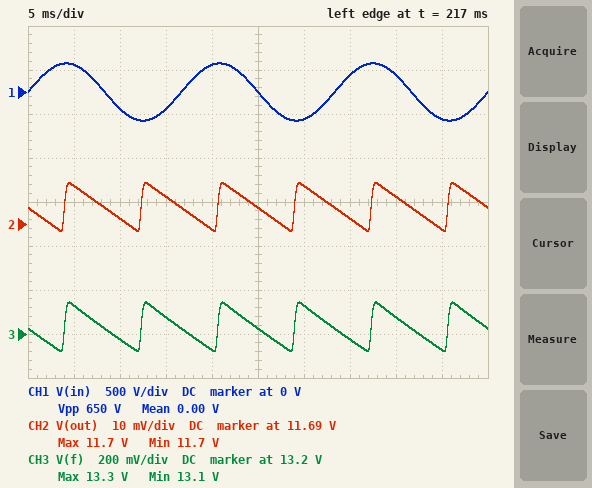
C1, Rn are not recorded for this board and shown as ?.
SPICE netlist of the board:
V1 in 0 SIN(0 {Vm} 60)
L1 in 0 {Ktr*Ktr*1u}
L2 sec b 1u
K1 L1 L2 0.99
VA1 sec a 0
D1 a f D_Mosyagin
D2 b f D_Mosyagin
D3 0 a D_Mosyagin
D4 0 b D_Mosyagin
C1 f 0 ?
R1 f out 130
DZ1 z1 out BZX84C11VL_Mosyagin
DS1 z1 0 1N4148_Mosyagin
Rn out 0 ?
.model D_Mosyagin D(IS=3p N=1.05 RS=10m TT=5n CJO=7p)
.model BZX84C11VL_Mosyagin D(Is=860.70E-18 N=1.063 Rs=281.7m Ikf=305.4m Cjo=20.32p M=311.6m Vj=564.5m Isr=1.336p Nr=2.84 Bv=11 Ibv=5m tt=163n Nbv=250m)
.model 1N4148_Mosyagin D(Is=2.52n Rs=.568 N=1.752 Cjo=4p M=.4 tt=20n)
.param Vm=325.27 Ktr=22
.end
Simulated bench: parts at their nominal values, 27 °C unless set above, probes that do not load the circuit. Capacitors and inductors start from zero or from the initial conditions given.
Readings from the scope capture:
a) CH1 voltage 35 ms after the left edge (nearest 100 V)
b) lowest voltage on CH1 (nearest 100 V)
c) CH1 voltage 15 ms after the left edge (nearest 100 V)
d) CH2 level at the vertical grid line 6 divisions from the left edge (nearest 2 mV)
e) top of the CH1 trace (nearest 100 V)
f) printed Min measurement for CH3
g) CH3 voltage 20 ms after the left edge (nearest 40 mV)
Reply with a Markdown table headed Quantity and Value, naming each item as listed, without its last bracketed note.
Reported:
| Quantity | Value |
|---|---|
| CH1 voltage 35 ms after the left edge | 200 V |
| lowest voltage on CH1 | -300 V |
| CH1 voltage 15 ms after the left edge | -200 V |
| CH2 level at the vertical grid line 6 divisions from the left edge | 11.698 V |
| top of the CH1 trace | 300 V |
| printed Min measurement for CH3 | 13.1 V |
| CH3 voltage 20 ms after the left edge | 13.12 V |
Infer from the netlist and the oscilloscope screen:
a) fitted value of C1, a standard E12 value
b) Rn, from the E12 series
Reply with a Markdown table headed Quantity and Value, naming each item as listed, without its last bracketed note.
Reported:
| Quantity | Value |
|---|---|
| fitted value of C1, a standard E12 value | 390 µF |
| Rn, from the E12 series | 3.9 kΩ |
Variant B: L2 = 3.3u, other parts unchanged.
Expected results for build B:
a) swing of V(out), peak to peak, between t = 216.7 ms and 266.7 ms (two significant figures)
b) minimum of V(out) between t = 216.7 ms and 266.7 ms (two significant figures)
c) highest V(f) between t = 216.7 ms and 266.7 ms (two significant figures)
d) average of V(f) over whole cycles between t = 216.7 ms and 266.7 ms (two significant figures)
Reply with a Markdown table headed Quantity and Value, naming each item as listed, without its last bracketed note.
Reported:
| Quantity | Value |
|---|---|
| swing of V(out), peak to peak, between t = 216.7 ms and 266.7 ms | 19 mV |
| minimum of V(out) between t = 216.7 ms and 266.7 ms | 12 V |
| highest V(f) between t = 216.7 ms and 266.7 ms | 25 V |
| average of V(f) over whole cycles between t = 216.7 ms and 266.7 ms | 24 V |
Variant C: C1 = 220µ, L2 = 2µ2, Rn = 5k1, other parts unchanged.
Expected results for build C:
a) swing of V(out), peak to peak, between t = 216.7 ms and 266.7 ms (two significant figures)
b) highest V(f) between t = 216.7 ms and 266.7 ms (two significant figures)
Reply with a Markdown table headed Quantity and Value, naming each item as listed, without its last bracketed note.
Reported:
| Quantity | Value |
|---|---|
| swing of V(out), peak to peak, between t = 216.7 ms and 266.7 ms | 25 mV |
| highest V(f) between t = 216.7 ms and 266.7 ms | 20 V |
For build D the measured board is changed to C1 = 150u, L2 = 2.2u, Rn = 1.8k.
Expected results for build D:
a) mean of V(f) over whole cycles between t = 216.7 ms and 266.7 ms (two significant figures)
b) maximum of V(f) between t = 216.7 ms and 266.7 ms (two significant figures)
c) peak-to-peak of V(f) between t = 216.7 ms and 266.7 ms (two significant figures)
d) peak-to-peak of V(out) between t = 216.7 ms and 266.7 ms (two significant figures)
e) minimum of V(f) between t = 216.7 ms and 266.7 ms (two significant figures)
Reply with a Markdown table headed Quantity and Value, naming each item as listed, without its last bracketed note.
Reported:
| Quantity | Value |
|---|---|
| mean of V(f) over whole cycles between t = 216.7 ms and 266.7 ms | 19 V |
| maximum of V(f) between t = 216.7 ms and 266.7 ms | 20 V |
| peak-to-peak of V(f) between t = 216.7 ms and 266.7 ms | 2.5 V |
| peak-to-peak of V(out) between t = 216.7 ms and 266.7 ms | 36 mV |
| minimum of V(f) between t = 216.7 ms and 266.7 ms | 18 V |
